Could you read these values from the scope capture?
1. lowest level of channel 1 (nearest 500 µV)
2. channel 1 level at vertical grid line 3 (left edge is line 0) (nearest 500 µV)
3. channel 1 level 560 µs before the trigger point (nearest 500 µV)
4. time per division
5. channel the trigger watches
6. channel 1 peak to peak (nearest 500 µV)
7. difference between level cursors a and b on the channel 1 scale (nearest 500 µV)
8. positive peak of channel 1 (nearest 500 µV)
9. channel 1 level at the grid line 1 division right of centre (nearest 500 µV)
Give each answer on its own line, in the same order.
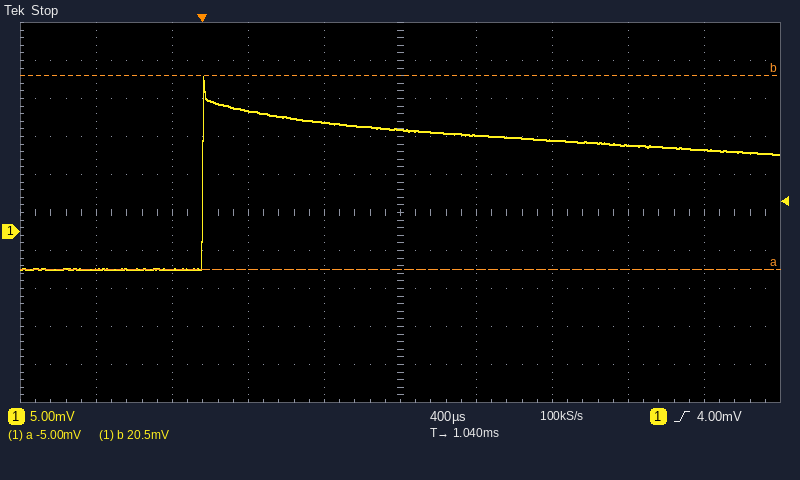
-5.0 mV
16.0 mV
-5.0 mV
400 µs
channel 1
25.5 mV
25.5 mV
20.5 mV
12.5 mV
